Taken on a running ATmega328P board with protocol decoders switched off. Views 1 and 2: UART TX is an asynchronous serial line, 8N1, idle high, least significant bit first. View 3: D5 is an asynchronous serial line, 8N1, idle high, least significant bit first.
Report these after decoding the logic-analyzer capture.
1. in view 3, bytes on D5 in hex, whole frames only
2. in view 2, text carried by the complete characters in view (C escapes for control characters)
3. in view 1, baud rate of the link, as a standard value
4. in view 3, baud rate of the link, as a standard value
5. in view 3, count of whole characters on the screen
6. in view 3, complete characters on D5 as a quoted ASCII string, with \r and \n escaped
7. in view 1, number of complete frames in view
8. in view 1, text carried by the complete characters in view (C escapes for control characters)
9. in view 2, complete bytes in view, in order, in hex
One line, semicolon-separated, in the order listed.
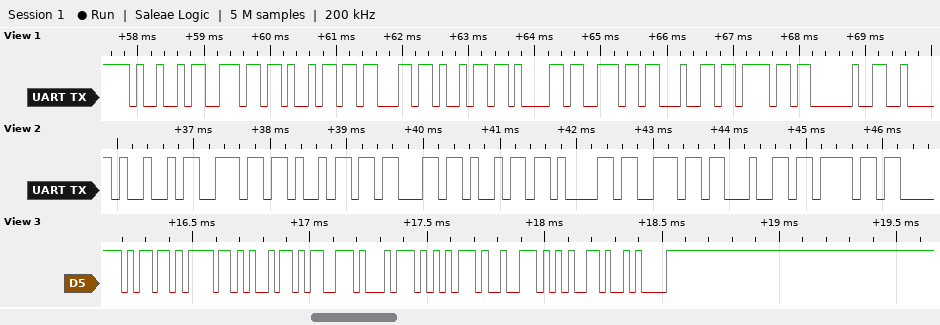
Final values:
6D 6F 69 73 74 75 72 65 0A; "Iniciando"; 9600 baud; 38400 baud; 9; "moisture\n"; 10; "Iniciando "; 49 6E 69 63 69 61 6E 64 6F
